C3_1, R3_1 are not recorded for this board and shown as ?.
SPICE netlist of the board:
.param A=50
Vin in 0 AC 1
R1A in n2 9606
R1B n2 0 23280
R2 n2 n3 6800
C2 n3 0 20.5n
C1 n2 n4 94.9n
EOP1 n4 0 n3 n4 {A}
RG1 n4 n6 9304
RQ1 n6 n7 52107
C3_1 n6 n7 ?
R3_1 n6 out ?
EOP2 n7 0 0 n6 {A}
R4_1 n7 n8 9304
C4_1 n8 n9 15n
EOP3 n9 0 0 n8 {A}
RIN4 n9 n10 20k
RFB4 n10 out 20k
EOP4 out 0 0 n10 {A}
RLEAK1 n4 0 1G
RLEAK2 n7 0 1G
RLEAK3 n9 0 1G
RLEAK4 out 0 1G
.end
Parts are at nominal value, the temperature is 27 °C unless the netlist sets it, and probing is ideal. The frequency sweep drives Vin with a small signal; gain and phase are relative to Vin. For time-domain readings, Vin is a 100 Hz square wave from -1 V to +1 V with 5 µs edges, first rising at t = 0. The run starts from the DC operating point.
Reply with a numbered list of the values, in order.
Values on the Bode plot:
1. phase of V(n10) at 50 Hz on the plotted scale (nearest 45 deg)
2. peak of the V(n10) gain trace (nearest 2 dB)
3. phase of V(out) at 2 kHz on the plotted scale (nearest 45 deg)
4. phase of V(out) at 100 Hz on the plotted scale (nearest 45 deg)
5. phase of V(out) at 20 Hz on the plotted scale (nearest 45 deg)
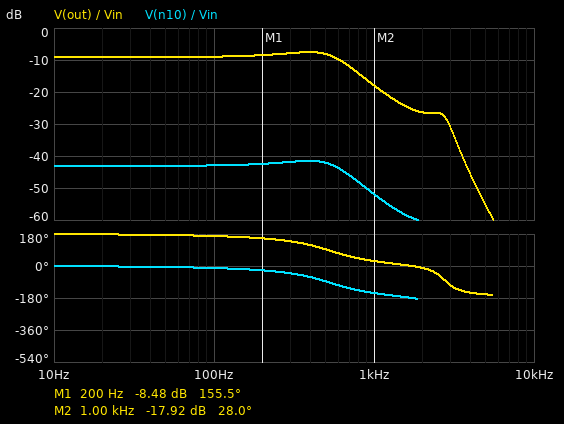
1. 0 deg
2. -42 dB
3. 0 deg
4. 180 deg
5. 180 deg
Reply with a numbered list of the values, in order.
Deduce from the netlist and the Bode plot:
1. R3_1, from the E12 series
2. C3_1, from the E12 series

1. 4.7 kΩ
2. 4.7 nF
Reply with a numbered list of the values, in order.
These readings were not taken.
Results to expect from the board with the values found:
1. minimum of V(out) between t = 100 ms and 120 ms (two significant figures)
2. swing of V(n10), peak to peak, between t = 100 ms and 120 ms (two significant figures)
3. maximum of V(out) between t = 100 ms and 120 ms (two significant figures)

1. -480 mV
2. 19 mV
3. 480 mV
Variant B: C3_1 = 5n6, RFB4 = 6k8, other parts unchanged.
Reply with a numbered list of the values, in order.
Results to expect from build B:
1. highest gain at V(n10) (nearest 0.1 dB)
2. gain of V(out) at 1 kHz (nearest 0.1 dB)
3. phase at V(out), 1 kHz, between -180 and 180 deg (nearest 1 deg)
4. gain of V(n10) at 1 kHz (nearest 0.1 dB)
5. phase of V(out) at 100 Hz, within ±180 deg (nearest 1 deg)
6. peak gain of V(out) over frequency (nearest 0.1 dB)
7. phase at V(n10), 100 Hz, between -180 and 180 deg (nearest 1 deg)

1. -41.2 dB
2. -15.3 dB
3. 4 deg
4. -49.3 dB
5. 167 deg
6. -7.2 dB
7. -13 deg
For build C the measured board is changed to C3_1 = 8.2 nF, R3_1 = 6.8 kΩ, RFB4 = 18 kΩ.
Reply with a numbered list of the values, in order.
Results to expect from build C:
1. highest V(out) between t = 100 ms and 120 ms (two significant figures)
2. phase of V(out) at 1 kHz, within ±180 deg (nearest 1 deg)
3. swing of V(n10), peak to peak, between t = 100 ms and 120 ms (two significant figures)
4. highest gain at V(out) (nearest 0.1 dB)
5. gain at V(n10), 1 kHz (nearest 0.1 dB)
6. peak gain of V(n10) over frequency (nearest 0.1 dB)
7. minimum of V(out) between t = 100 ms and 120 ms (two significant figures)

1. 710 mV
2. 20 deg
3. 28 mV
4. -4.0 dB
5. -46.2 dB
6. -38.0 dB
7. -710 mV
